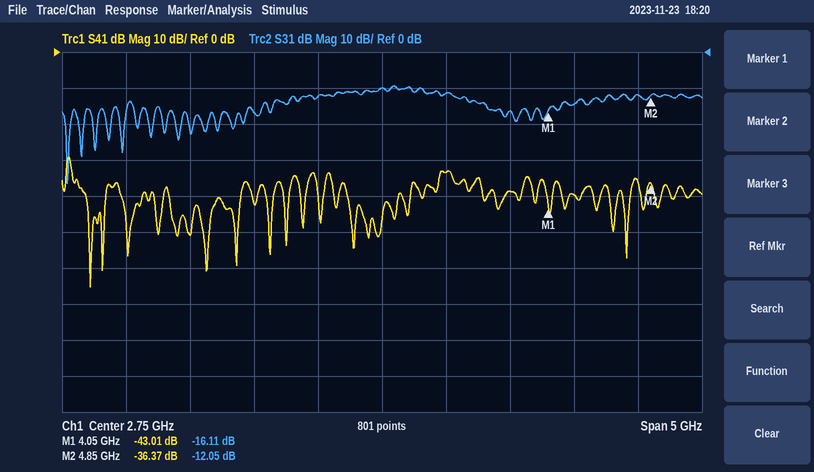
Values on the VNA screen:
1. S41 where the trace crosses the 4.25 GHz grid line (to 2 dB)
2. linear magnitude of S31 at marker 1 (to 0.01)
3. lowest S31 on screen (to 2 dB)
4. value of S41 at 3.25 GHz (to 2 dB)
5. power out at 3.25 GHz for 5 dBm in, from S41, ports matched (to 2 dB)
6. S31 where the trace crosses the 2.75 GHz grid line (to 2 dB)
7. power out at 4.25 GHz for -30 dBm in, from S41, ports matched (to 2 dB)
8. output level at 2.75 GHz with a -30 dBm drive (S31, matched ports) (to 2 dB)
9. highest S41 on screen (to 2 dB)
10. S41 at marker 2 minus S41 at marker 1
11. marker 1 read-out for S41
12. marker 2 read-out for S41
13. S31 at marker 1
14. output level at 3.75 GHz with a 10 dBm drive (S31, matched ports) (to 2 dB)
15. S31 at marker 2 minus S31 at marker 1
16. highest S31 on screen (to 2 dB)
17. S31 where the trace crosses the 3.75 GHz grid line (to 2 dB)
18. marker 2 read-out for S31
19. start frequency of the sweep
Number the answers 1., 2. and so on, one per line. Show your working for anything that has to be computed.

1. -40 dB
2. 10^(-16.11/20) ≈ 0.16
3. -36 dB
4. -34 dB
5. 5 dBm + (-34 dB) = -28 dBm
6. -10 dB
7. -30 dBm + (-40 dB) = -70 dBm
8. -30 dBm + (-10 dB) = -40 dBm
9. -30 dB
10. -36.37 − (-43.01) = 6.64 dB
11. -43.01 dB
12. -36.37 dB
13. -16.11 dB
14. 10 dBm + (-16 dB) = -6 dBm
15. -12.05 − (-16.11) = 4.06 dB
16. -10 dB
17. -16 dB
18. -12.05 dB
19. 250 MHz
